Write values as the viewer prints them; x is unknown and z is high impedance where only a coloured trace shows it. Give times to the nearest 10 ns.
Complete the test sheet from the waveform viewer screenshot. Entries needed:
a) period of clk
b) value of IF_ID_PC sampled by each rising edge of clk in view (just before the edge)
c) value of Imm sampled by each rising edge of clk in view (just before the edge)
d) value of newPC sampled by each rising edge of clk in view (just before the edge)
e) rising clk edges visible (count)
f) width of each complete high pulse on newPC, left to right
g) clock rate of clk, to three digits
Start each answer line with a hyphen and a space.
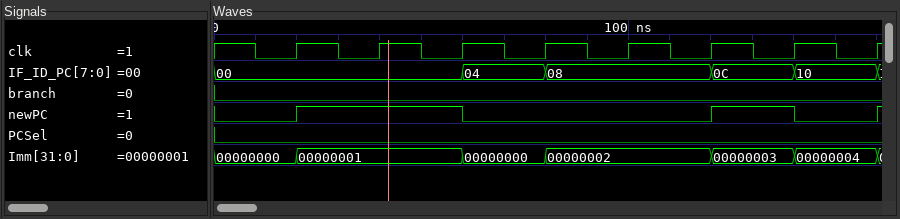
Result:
- 20 ns
- 00, 00, 00, 04, 08, 08, 0C, 10
- 00000000, 00000001, 00000001, 00000000, 00000002, 00000002, 00000003, 00000004
- 0 1 1 0 0 0 1 0
- 8
- 40 ns, 20 ns
- 50.0 MHz
